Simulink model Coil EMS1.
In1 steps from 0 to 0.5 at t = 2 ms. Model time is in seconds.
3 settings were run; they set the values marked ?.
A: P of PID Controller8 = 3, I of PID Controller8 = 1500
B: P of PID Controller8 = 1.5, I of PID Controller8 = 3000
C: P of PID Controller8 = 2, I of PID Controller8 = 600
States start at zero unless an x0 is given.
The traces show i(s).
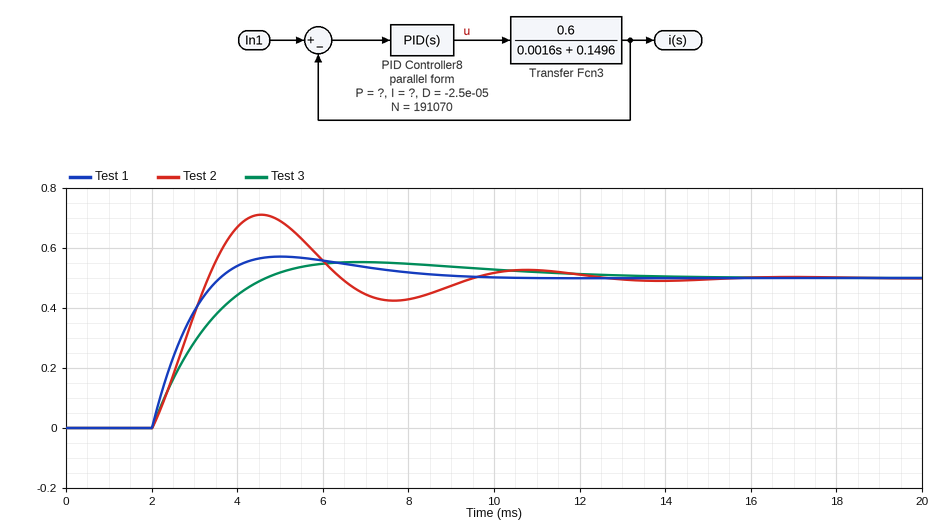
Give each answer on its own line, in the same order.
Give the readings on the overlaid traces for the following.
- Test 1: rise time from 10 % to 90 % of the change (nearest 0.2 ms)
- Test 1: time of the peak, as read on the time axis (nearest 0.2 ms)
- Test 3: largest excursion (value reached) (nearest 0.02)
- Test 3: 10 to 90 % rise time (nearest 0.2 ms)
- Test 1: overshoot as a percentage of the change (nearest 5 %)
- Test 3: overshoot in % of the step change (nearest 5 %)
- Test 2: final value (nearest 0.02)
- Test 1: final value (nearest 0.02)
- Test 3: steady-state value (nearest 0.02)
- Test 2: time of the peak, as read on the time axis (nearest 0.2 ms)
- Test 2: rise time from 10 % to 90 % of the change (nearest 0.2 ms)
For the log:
1.2 ms
5.0 ms
0.56
2.0 ms
15 %
10 %
0.50
0.50
0.50
4.6 ms
1.0 ms
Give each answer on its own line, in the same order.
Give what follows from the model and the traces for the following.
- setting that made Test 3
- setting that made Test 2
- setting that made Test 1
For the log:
C
B
A
